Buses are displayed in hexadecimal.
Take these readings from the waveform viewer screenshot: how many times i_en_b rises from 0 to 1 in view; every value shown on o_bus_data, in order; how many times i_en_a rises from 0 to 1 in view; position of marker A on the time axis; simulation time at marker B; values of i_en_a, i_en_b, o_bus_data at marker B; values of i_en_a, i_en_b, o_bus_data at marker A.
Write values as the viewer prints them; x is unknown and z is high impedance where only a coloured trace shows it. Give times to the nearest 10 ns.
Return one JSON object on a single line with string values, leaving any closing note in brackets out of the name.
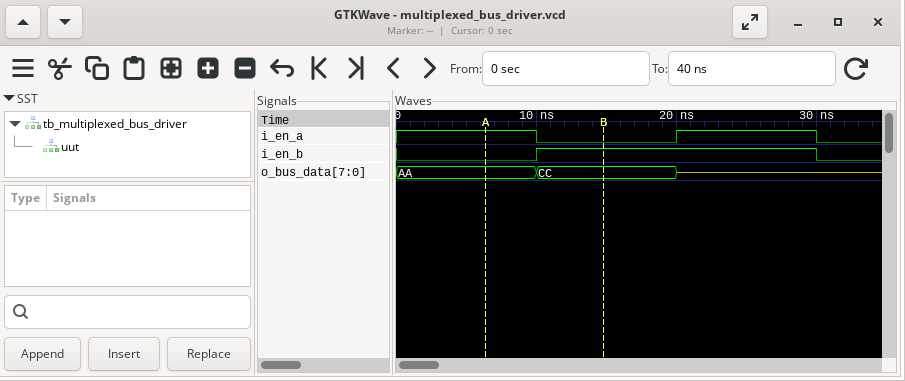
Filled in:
{"how many times i_en_b rises from 0 to 1 in view": "1", "every value shown on o_bus_data, in order": "AA, CC, z", "how many times i_en_a rises from 0 to 1 in view": "1", "position of marker A on the time axis": "10 ns", "simulation time at marker B": "10 ns", "values of i_en_a, i_en_b, o_bus_data at marker B": "i_en_a=0, i_en_b=1, o_bus_data=CC", "values of i_en_a, i_en_b, o_bus_data at marker A": "i_en_a=1, i_en_b=0, o_bus_data=AA"}
